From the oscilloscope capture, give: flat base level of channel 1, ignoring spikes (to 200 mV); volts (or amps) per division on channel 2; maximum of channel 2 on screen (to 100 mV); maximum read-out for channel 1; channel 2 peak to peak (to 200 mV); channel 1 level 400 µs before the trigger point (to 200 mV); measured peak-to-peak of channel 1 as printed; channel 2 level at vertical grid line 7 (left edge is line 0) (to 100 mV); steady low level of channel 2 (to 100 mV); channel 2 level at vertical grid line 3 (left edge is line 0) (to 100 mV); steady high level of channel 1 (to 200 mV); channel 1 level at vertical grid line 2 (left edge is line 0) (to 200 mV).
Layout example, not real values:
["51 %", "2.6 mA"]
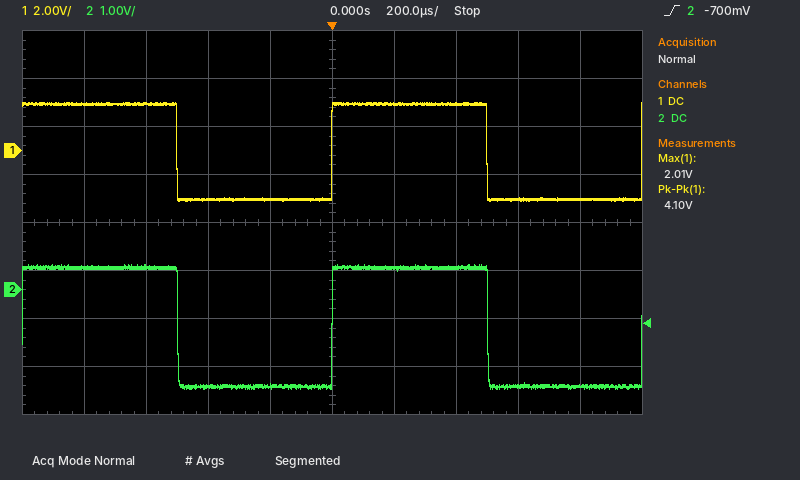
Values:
["-2.0 V", "1 V", "500 mV", "2.01 V", "2.6 V", "-2.0 V", "4.10 V", "500 mV", "-2.0 V", "-2.0 V", "2.0 V", "2.0 V"]
